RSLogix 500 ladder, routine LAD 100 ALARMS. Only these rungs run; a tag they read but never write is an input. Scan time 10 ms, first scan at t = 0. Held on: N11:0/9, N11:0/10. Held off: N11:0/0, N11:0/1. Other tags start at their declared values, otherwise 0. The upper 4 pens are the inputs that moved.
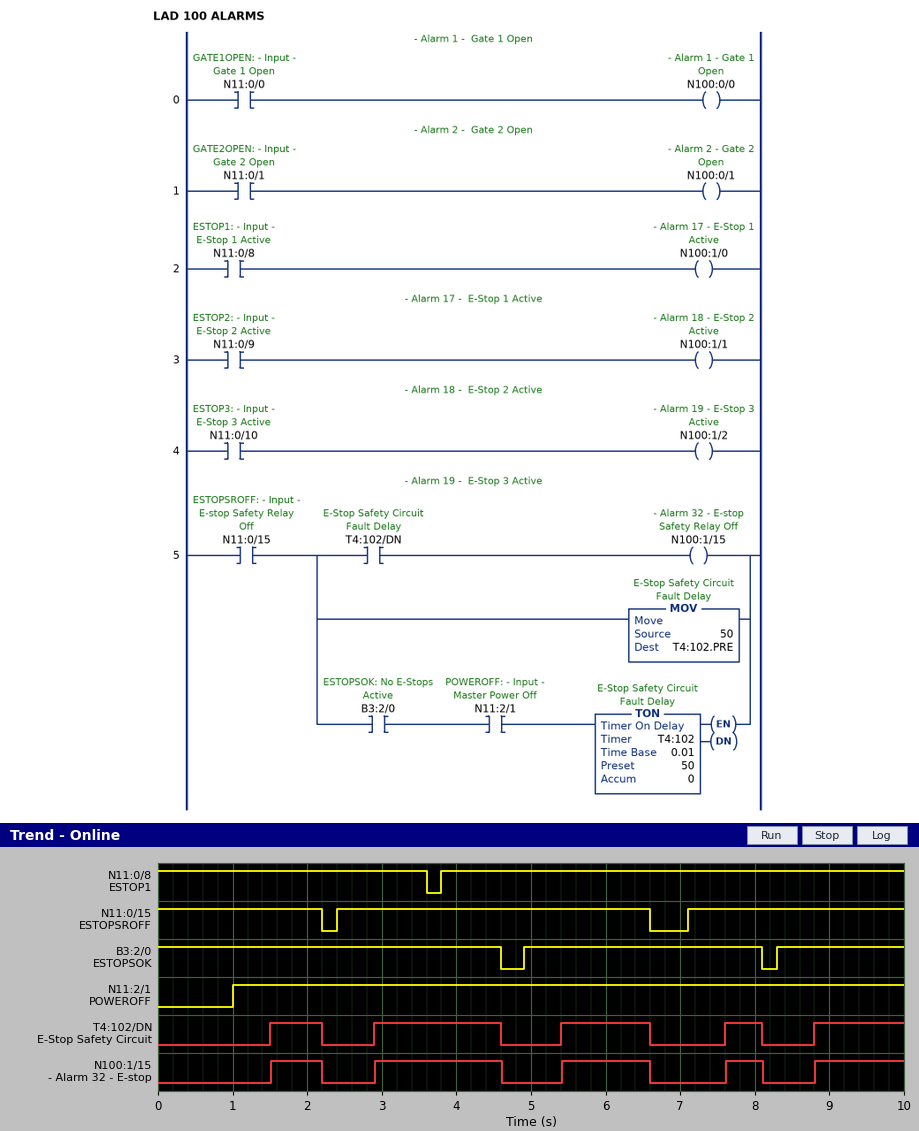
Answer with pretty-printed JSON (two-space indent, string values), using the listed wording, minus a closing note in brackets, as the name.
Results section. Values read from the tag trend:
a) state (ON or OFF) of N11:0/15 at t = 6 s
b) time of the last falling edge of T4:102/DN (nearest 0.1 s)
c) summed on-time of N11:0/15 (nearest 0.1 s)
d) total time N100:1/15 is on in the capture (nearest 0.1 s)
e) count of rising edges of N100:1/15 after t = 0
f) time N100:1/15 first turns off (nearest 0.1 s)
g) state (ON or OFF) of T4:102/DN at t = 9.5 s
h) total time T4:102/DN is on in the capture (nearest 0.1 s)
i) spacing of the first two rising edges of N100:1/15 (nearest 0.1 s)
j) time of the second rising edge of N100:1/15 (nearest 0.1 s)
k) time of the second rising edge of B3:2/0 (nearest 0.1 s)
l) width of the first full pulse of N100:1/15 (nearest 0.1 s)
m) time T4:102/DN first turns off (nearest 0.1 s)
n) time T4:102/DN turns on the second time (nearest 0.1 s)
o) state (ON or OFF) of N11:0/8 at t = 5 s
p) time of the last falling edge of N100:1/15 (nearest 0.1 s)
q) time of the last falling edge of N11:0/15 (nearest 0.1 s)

{
  "state (ON or OFF) of N11:0/15 at t = 6 s": "ON",
  "time of the last falling edge of T4:102/DN": "8.1 s",
  "summed on-time of N11:0/15": "9.3 s",
  "total time N100:1/15 is on in the capture": "5.3 s",
  "count of rising edges of N100:1/15 after t = 0": "5",
  "time N100:1/15 first turns off": "2.2 s",
  "state (ON or OFF) of T4:102/DN at t = 9.5 s": "ON",
  "total time T4:102/DN is on in the capture": "5.3 s",
  "spacing of the first two rising edges of N100:1/15": "1.4 s",
  "time of the second rising edge of N100:1/15": "2.9 s",
  "time of the second rising edge of B3:2/0": "8.3 s",
  "width of the first full pulse of N100:1/15": "0.7 s",
  "time T4:102/DN first turns off": "2.2 s",
  "time T4:102/DN turns on the second time": "2.9 s",
  "state (ON or OFF) of N11:0/8 at t = 5 s": "ON",
  "time of the last falling edge of N100:1/15": "8.1 s",
  "time of the last falling edge of N11:0/15": "6.6 s"
}
